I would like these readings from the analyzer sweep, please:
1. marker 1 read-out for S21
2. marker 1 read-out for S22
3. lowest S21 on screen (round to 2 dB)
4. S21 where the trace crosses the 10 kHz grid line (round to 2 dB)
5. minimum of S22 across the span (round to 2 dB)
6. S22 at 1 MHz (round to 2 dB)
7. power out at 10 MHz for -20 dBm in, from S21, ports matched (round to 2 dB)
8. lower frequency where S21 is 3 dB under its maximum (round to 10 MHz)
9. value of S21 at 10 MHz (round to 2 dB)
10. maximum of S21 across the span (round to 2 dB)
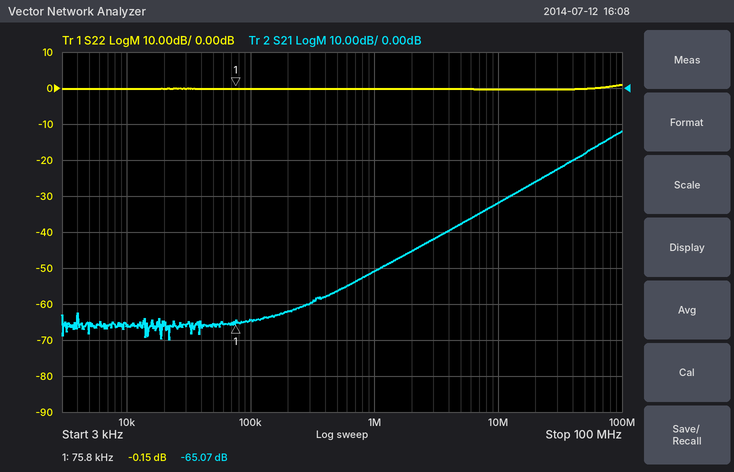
-65.07 dB
-0.15 dB
-70 dB
-66 dB
0 dB
0 dB
-52 dBm
70 MHz
-32 dB
-12 dB
